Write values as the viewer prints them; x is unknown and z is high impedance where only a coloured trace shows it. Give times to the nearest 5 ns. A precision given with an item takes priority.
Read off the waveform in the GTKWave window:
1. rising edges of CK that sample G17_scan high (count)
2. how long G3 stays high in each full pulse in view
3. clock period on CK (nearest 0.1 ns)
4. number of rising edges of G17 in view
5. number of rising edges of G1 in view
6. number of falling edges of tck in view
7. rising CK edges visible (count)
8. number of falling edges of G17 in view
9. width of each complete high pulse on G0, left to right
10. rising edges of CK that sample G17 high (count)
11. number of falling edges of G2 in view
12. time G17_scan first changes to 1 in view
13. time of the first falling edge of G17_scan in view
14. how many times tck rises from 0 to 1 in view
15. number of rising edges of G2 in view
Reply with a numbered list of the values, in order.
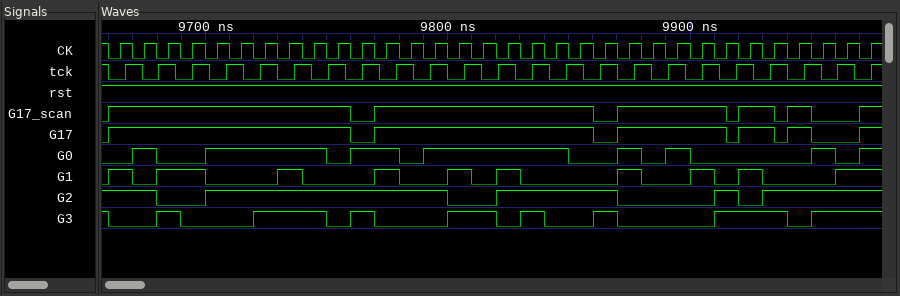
1. 28
2. 10 ns, 30 ns, 10 ns, 20 ns, 10 ns, 10 ns, 30 ns
3. 10 ns
4. 6
5. 10
6. 23
7. 32
8. 5
9. 10 ns, 50 ns, 20 ns, 60 ns, 10 ns, 10 ns, 10 ns
10. 28
11. 4
12. 9660 ns
13. 9760 ns
14. 23
15. 4
